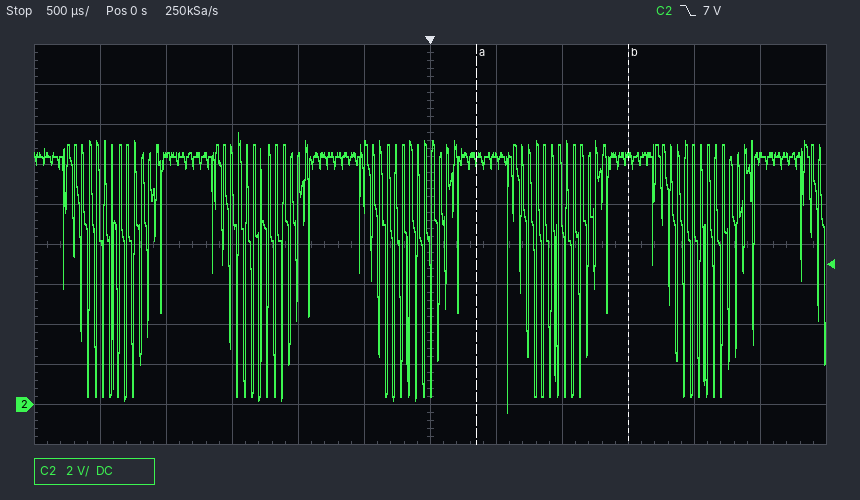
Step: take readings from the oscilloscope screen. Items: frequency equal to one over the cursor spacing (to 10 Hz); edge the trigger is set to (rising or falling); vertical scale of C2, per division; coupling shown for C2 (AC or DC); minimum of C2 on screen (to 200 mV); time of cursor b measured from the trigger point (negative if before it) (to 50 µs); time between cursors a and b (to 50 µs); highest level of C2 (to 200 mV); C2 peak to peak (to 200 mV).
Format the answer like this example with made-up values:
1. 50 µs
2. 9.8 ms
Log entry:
1. 870 Hz
2. falling
3. 2 V
4. DC
5. -400 mV
6. +1.50 ms
7. 1.15 ms
8. 13.6 V
9. 14.0 V
